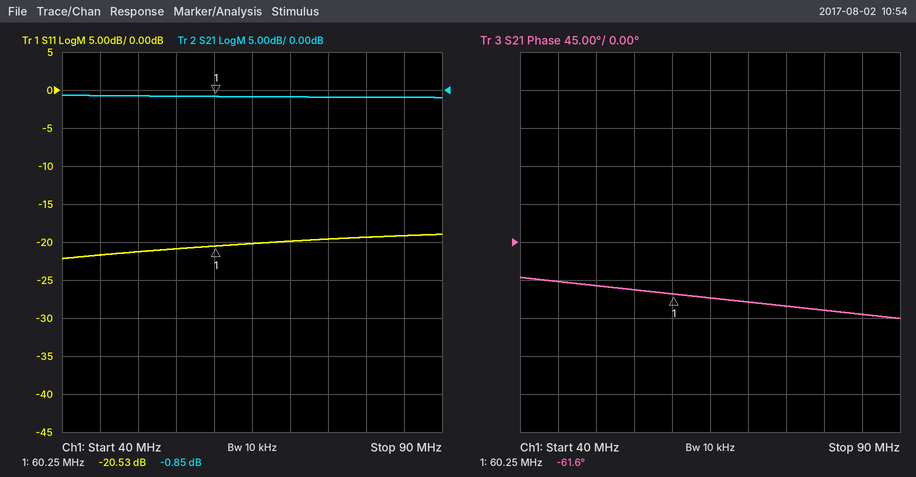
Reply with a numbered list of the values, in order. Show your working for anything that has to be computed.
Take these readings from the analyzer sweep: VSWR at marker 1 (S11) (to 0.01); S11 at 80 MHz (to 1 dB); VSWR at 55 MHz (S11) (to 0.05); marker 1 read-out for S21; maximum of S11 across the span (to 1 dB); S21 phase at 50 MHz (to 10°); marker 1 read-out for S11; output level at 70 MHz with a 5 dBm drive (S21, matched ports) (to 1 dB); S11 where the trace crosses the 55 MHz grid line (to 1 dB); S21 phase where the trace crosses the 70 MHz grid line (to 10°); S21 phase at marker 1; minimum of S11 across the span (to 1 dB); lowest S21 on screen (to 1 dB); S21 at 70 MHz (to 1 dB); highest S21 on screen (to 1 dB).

1. (1 + 0.0941)/(1 − 0.0941) ≈ 1.21
2. -19 dB
3. |Γ| = 10^(-21/20) = 0.0891; VSWR = (1 + 0.0891)/(1 − 0.0891) ≈ 1.20
4. -0.85 dB
5. -19 dB
6. -50°
7. -20.53 dB
8. 5 dBm + (-1 dB) = 4 dBm
9. -21 dB
10. -70°
11. -61.6°
12. -22 dB
13. -1 dB
14. -1 dB
15. -1 dB
